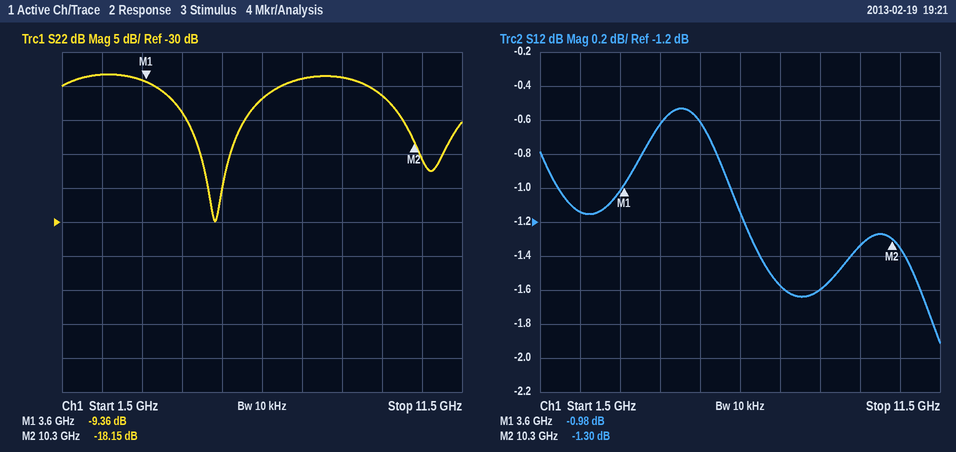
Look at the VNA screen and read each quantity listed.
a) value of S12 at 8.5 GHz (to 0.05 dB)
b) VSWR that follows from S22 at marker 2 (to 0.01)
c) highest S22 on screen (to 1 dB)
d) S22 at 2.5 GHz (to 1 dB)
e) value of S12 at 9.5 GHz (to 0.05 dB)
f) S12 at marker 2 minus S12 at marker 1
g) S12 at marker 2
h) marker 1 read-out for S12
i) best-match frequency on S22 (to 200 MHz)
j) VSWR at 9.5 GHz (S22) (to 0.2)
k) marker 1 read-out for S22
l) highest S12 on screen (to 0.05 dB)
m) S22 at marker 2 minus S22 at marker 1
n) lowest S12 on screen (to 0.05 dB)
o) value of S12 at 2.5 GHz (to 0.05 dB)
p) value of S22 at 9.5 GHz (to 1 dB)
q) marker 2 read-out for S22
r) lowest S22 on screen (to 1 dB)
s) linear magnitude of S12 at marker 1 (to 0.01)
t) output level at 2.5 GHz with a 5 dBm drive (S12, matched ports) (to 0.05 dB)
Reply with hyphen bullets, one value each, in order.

- -1.60 dB
- 1.28
- -8 dB
- -8 dB
- -1.35 dB
- -0.32 dB
- -1.30 dB
- -0.98 dB
- 5.4 GHz
- 1.8
- -9.36 dB
- -0.55 dB
- -8.79 dB
- -1.90 dB
- -1.15 dB
- -11 dB
- -18.15 dB
- -30 dB
- 0.89
- 3.85 dBm
